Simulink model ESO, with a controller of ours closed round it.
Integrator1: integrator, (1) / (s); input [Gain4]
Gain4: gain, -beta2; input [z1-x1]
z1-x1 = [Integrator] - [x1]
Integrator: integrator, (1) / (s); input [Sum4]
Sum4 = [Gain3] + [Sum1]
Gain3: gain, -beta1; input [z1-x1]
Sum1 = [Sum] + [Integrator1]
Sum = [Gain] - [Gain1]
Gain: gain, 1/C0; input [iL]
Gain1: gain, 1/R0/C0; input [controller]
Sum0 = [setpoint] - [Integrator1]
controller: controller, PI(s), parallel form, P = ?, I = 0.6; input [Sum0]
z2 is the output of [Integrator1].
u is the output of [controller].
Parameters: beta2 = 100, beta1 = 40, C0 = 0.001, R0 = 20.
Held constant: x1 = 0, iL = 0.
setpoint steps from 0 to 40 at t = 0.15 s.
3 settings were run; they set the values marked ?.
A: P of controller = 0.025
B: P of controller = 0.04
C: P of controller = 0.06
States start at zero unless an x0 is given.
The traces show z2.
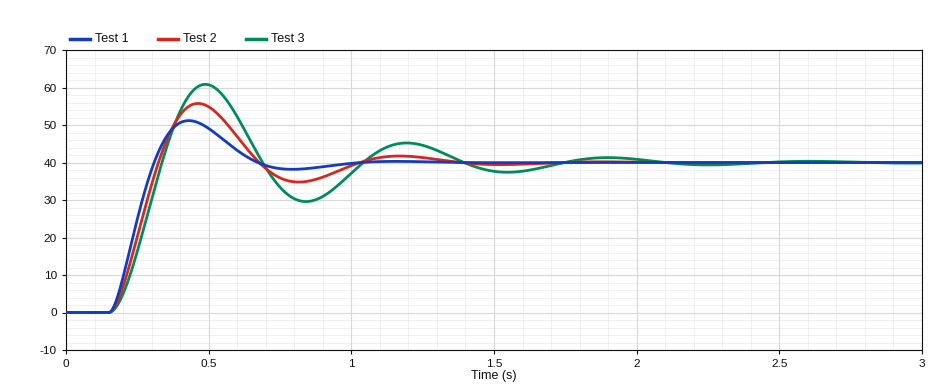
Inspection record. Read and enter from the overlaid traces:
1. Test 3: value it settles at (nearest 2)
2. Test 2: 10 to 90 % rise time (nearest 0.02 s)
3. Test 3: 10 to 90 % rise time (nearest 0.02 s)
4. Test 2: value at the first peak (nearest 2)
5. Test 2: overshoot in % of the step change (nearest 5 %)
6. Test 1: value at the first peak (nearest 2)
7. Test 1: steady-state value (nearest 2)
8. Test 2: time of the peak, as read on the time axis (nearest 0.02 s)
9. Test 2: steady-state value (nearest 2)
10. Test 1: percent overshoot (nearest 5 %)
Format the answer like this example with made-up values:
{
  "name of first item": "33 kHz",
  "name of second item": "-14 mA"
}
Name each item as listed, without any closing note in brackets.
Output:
{
  "Test 3: value it settles at": "40",
  "Test 2: 10 to 90 % rise time": "0.12 s",
  "Test 3: 10 to 90 % rise time": "0.12 s",
  "Test 2: value at the first peak": "56",
  "Test 2: overshoot in % of the step change": "40 %",
  "Test 1: value at the first peak": "52",
  "Test 1: steady-state value": "40",
  "Test 2: time of the peak, as read on the time axis": "0.46 s",
  "Test 2: steady-state value": "40",
  "Test 1: percent overshoot": "30 %"
}
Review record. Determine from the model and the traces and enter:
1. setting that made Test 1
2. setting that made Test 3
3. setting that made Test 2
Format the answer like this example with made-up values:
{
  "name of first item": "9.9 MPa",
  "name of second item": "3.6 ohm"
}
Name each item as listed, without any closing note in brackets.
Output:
{
  "setting that made Test 1": "C",
  "setting that made Test 3": "A",
  "setting that made Test 2": "B"
}
